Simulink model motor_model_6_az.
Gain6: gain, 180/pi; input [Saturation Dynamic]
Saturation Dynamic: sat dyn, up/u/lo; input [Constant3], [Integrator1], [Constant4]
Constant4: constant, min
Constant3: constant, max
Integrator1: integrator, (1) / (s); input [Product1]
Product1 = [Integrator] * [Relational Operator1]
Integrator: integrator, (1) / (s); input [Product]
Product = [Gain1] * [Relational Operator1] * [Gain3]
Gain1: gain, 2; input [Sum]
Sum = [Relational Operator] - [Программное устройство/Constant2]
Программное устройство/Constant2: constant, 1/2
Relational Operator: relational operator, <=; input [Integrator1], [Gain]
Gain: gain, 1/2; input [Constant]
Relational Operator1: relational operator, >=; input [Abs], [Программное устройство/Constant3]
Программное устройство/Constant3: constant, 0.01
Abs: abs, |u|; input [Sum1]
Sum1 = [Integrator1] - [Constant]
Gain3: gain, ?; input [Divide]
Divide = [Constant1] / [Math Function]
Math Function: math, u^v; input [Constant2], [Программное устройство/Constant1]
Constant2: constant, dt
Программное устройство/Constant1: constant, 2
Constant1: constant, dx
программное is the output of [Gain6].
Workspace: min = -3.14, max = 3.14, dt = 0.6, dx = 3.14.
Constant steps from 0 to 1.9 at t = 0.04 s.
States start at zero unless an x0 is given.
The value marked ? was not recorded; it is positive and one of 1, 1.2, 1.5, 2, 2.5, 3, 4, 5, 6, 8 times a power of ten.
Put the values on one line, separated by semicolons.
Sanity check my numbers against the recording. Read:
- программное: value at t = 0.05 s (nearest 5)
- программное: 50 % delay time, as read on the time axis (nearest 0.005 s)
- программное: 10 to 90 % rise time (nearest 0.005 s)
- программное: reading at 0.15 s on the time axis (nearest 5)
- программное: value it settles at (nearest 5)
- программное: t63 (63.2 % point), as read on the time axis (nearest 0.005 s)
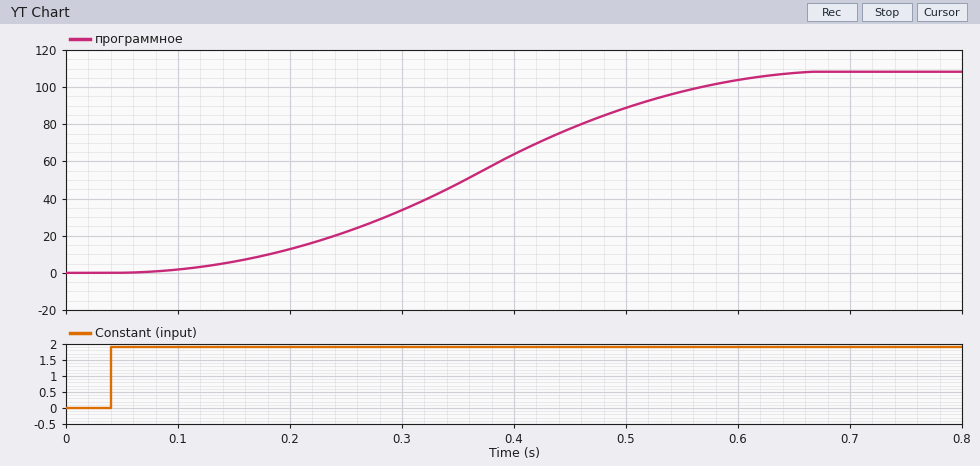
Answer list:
0; 0.370 s; 0.360 s; 5; 110; 0.415 s
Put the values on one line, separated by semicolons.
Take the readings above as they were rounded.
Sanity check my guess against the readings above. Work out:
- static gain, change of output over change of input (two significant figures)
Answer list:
58
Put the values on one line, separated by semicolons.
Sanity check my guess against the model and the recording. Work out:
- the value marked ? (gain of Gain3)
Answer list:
2
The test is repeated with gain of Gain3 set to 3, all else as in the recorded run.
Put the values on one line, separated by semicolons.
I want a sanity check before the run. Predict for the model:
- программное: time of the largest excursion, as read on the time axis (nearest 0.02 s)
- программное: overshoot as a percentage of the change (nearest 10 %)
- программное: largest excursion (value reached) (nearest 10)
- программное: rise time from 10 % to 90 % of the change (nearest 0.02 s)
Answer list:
0.56 s; 40 %; 110; 0.20 s
